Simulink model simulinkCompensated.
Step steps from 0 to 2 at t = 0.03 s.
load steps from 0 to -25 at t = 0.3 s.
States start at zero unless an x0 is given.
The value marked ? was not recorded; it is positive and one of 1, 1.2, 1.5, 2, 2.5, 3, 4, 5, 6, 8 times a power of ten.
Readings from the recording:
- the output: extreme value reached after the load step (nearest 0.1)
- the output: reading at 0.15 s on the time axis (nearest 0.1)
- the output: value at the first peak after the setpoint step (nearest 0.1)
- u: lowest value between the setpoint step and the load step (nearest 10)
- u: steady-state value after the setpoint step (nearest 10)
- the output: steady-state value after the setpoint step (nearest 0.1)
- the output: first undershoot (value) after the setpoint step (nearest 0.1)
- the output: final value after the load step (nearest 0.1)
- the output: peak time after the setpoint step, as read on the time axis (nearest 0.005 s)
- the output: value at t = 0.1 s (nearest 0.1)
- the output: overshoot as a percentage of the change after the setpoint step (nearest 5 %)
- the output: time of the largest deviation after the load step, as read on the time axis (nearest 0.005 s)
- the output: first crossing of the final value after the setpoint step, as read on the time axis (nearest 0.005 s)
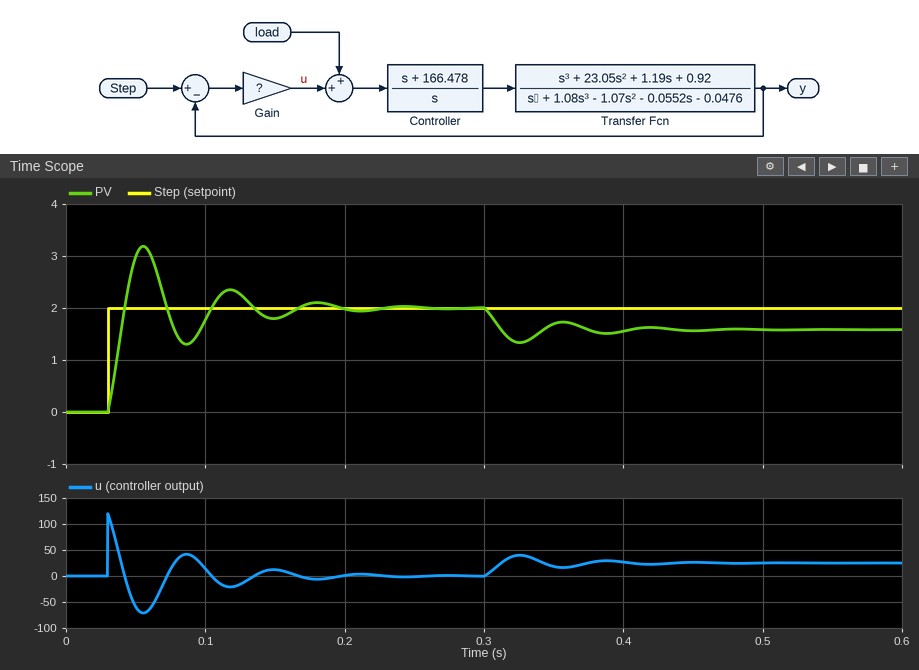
1.3
1.8
3.2
-70
0
2.0
1.3
1.6
0.055 s
1.8
60 %
0.325 s
0.040 s
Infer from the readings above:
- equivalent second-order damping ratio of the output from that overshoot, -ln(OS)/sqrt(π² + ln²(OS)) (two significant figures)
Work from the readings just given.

0.16
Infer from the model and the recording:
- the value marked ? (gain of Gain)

60
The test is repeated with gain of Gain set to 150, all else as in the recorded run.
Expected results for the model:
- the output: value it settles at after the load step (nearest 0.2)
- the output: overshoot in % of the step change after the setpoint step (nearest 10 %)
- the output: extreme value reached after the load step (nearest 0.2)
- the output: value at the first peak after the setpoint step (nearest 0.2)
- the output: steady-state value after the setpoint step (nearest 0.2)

1.8
40 %
1.8
2.8
2.0
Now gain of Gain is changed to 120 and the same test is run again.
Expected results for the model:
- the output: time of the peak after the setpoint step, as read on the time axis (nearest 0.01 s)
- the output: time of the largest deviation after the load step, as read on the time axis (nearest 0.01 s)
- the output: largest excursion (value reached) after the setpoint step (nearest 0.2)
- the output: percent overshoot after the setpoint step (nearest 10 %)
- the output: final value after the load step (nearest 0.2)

0.05 s
0.32 s
2.8
40 %
1.8
